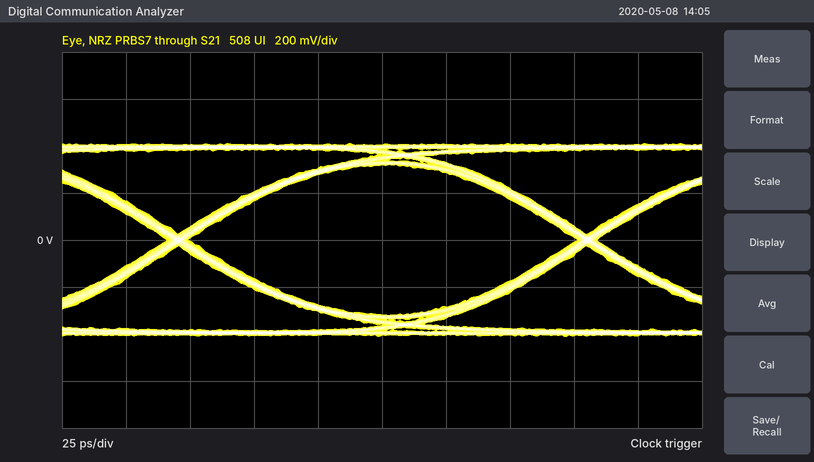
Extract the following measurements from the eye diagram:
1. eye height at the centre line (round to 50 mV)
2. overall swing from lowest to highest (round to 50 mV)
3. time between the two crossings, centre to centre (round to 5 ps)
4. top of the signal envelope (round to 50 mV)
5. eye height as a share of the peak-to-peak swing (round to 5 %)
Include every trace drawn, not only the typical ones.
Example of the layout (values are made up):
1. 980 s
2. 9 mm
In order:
1. 650 mV
2. 800 mV
3. 160 ps
4. 400 mV
5. 80 %
